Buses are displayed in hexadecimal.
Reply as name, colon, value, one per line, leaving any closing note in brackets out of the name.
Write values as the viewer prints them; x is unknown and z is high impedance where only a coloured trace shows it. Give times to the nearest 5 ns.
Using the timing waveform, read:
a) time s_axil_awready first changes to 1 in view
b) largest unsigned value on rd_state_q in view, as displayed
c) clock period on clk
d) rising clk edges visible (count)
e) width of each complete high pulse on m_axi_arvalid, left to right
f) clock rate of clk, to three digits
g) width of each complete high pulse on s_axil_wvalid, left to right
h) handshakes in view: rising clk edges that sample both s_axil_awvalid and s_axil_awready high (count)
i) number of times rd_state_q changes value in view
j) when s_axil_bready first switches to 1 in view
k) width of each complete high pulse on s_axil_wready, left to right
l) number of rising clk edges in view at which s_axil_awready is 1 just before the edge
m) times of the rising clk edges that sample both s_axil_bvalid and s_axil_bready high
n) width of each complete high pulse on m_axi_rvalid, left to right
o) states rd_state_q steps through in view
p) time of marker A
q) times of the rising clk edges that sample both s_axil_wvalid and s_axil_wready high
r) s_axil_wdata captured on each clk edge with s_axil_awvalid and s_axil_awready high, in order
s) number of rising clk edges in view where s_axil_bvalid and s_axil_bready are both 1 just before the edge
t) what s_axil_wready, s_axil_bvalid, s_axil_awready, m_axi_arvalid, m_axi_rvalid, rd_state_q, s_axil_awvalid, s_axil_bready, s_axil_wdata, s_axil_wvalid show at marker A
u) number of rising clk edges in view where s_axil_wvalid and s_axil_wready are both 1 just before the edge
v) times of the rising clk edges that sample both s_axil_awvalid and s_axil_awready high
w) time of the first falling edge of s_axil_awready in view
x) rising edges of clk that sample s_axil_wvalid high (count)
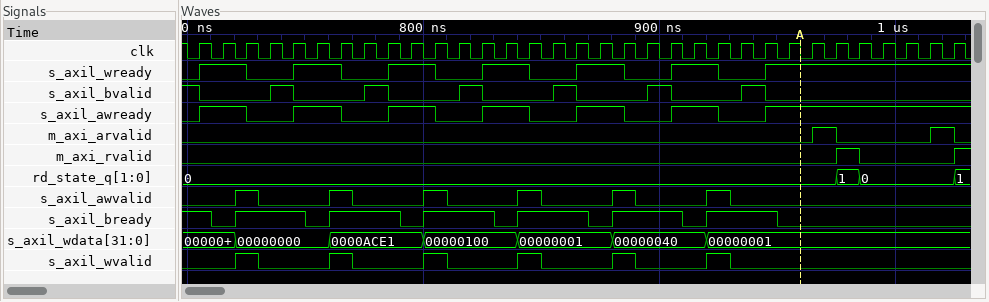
time s_axil_awready first changes to 1 in view: 705 ns
largest unsigned value on rd_state_q in view, as displayed: 1
clock period on clk: 10 ns
rising clk edges visible: 33
width of each complete high pulse on m_axi_arvalid, left to right: 10 ns, 10 ns
clock rate of clk, to three digits: 100 MHz
width of each complete high pulse on s_axil_wvalid, left to right: 10 ns, 10 ns, 10 ns, 10 ns, 10 ns, 10 ns
handshakes in view: rising clk edges that sample both s_axil_awvalid and s_axil_awready high: 6
number of times rd_state_q changes value in view: 3
when s_axil_bready first switches to 1 in view: 720 ns
width of each complete high pulse on s_axil_wready, left to right: 20 ns, 20 ns, 20 ns, 20 ns, 20 ns, 20 ns
number of rising clk edges in view at which s_axil_awready is 1 just before the edge: 20
times of the rising clk edges that sample both s_axil_bvalid and s_axil_bready high: 705 ns, 745 ns, 785 ns, 825 ns, 865 ns, 905 ns, 945 ns
width of each complete high pulse on m_axi_rvalid, left to right: 10 ns
states rd_state_q steps through in view: 0, 1, 0, 1
time of marker A: 960 ns
times of the rising clk edges that sample both s_axil_wvalid and s_axil_wready high: 725 ns, 765 ns, 805 ns, 845 ns, 885 ns, 925 ns
s_axil_wdata captured on each clk edge with s_axil_awvalid and s_axil_awready high, in order: 00000000, 0000ACE1, 00000100, 00000001, 00000040, 00000001
number of rising clk edges in view where s_axil_bvalid and s_axil_bready are both 1 just before the edge: 7
what s_axil_wready, s_axil_bvalid, s_axil_awready, m_axi_arvalid, m_axi_rvalid, rd_state_q, s_axil_awvalid, s_axil_bready, s_axil_wdata, s_axil_wvalid show at marker A: s_axil_wready=1, s_axil_bvalid=0, s_axil_awready=1, m_axi_arvalid=0, m_axi_rvalid=0, rd_state_q=0, s_axil_awvalid=0, s_axil_bready=0, s_axil_wdata=00000001, s_axil_wvalid=0
number of rising clk edges in view where s_axil_wvalid and s_axil_wready are both 1 just before the edge: 6
times of the rising clk edges that sample both s_axil_awvalid and s_axil_awready high: 725 ns, 765 ns, 805 ns, 845 ns, 885 ns, 925 ns
time of the first falling edge of s_axil_awready in view: 725 ns
rising edges of clk that sample s_axil_wvalid high: 6
